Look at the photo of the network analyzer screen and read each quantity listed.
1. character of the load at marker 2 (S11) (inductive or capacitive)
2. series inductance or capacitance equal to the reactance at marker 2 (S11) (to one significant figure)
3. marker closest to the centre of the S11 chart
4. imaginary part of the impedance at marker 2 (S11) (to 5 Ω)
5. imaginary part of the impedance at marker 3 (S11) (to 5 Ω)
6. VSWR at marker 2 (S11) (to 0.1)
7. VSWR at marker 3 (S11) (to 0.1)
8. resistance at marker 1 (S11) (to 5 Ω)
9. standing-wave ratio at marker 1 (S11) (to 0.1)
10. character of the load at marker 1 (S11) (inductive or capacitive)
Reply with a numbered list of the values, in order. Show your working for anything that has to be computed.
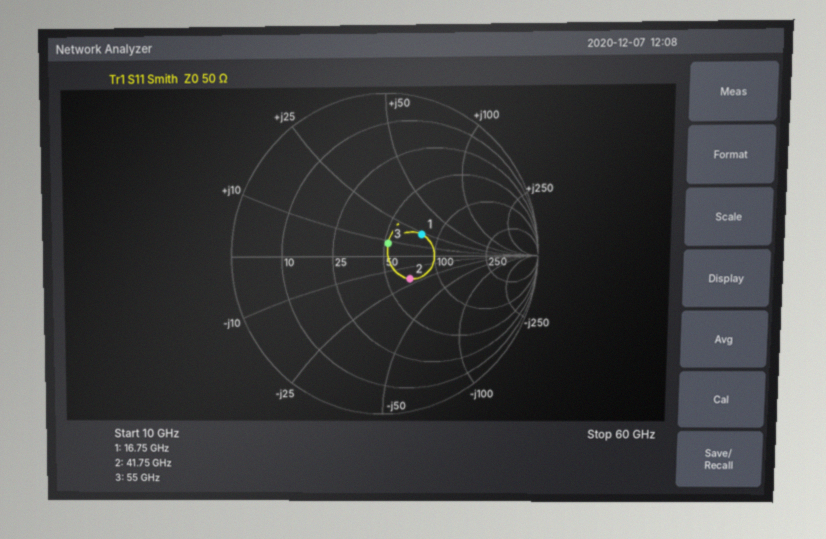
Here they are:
1. capacitive
2. C = 1/(2π × 41.75 GHz × 20 Ω) ≈ 191 fF, so 200 fF to one significant figure
3. marker 3
4. -20 Ω
5. +10 Ω
6. 1.6
7. 1.2
8. 80 Ω
9. 1.8
10. inductive
